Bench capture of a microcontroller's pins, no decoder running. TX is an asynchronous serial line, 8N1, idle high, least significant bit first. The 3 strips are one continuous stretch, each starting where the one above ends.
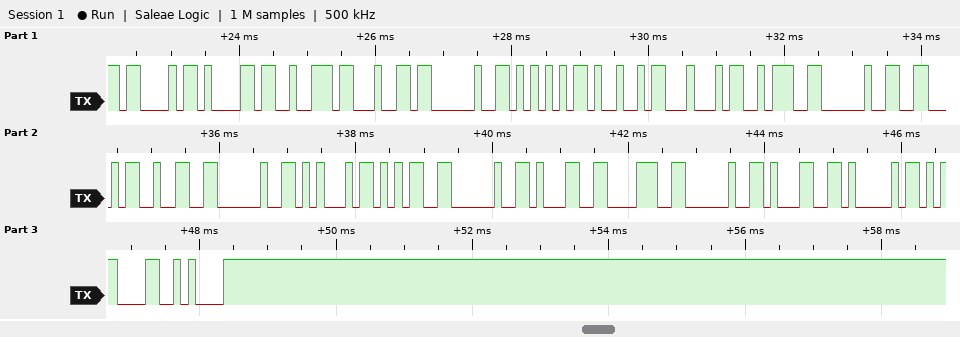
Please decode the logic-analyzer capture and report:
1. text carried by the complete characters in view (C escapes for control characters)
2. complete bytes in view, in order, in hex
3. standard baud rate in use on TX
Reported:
"Card UID: F2 E5 18 1A\r\n"
0x43 0x61 0x72 0x64 0x20 0x55 0x49 0x44 0x3A 0x20 0x46 0x32 0x20 0x45 0x35 0x20 0x31 0x38 0x20 0x31 0x41 0x0D 0x0A
9600 baud
